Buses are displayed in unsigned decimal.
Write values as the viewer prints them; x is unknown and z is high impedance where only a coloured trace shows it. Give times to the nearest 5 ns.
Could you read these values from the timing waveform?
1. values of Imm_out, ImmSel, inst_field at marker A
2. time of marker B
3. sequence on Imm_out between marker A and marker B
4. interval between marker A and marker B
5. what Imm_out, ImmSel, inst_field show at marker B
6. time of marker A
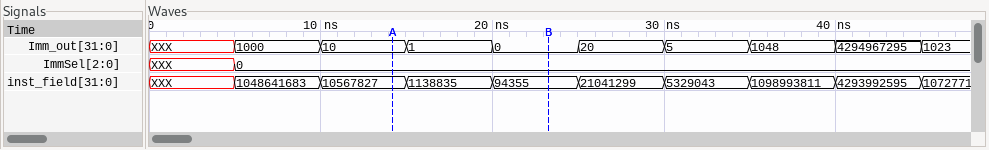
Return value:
Imm_out=10, ImmSel=0, inst_field=10567827
25 ns
10, 1, 0
10 ns
Imm_out=0, ImmSel=0, inst_field=94355
15 ns
